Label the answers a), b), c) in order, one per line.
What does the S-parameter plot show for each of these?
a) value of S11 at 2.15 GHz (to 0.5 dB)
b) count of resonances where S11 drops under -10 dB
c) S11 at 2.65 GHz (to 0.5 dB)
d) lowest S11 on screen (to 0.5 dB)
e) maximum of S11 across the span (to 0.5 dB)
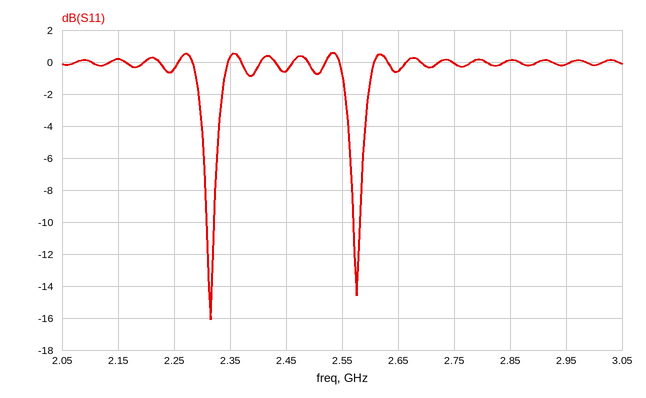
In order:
a) 0.0 dB
b) 2
c) -0.5 dB
d) -16.0 dB
e) 0.5 dB
